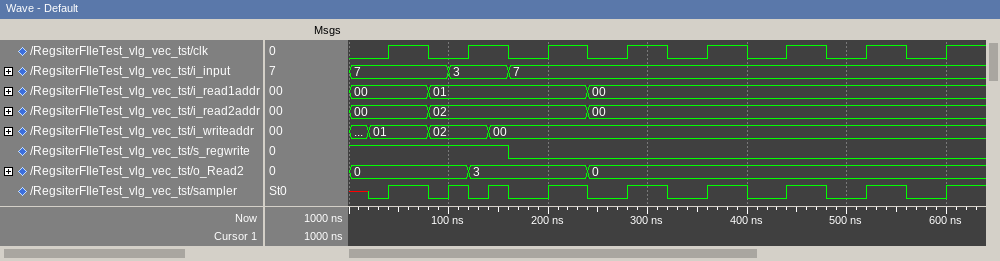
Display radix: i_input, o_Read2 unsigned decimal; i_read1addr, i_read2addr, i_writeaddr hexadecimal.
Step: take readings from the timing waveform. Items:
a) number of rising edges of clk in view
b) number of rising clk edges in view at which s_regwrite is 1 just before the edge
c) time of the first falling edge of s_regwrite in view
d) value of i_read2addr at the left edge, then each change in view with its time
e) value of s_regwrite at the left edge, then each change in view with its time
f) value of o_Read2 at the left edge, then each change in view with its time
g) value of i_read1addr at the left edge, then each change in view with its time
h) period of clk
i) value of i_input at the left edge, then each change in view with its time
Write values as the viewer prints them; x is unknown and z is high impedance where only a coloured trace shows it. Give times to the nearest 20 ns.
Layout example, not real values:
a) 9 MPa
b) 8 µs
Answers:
a) 8
b) 2
c) 160 ns
d) 00, 02 at 80 ns, 00 at 240 ns
e) 1, 0 at 160 ns
f) 0, 3 at 120 ns, 0 at 240 ns
g) 00, 01 at 80 ns, 00 at 240 ns
h) 80 ns
i) 7, 3 at 100 ns, 7 at 160 ns
